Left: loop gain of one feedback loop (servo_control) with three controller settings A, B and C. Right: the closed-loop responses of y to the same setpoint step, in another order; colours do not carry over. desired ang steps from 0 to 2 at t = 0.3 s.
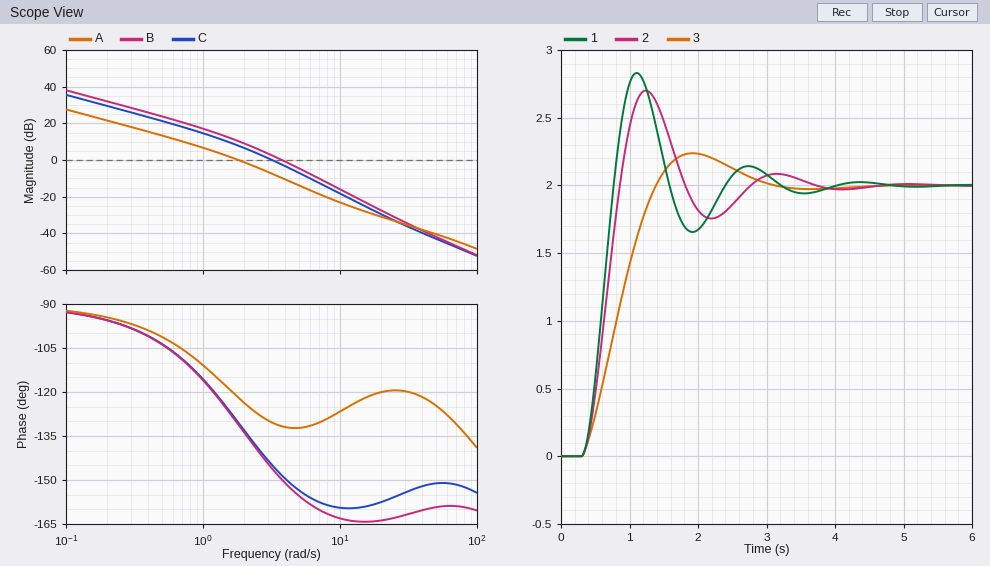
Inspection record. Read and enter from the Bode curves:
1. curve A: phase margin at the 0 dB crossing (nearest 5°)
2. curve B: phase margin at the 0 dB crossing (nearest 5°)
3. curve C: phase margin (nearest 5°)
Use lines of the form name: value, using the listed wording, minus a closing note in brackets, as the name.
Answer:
curve A: phase margin at the 0 dB crossing: 60°
curve B: phase margin at the 0 dB crossing: 30°
curve C: phase margin: 35°
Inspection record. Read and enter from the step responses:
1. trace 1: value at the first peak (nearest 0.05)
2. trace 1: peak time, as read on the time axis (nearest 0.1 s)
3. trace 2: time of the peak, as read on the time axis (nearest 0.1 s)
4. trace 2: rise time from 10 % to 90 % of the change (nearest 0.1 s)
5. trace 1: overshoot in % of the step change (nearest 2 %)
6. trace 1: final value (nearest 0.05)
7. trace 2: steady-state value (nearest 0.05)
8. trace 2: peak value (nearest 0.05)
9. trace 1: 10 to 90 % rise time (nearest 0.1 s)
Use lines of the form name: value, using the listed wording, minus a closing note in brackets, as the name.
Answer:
trace 1: value at the first peak: 2.85
trace 1: peak time, as read on the time axis: 1.1 s
trace 2: time of the peak, as read on the time axis: 1.2 s
trace 2: rise time from 10 % to 90 % of the change: 0.4 s
trace 1: overshoot in % of the step change: 42 %
trace 1: final value: 2.00
trace 2: steady-state value: 2.00
trace 2: peak value: 2.70
trace 1: 10 to 90 % rise time: 0.3 s
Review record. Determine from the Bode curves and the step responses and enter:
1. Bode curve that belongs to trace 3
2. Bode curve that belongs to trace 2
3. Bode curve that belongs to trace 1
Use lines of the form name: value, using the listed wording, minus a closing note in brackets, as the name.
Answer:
Bode curve that belongs to trace 3: A
Bode curve that belongs to trace 2: C
Bode curve that belongs to trace 1: B
